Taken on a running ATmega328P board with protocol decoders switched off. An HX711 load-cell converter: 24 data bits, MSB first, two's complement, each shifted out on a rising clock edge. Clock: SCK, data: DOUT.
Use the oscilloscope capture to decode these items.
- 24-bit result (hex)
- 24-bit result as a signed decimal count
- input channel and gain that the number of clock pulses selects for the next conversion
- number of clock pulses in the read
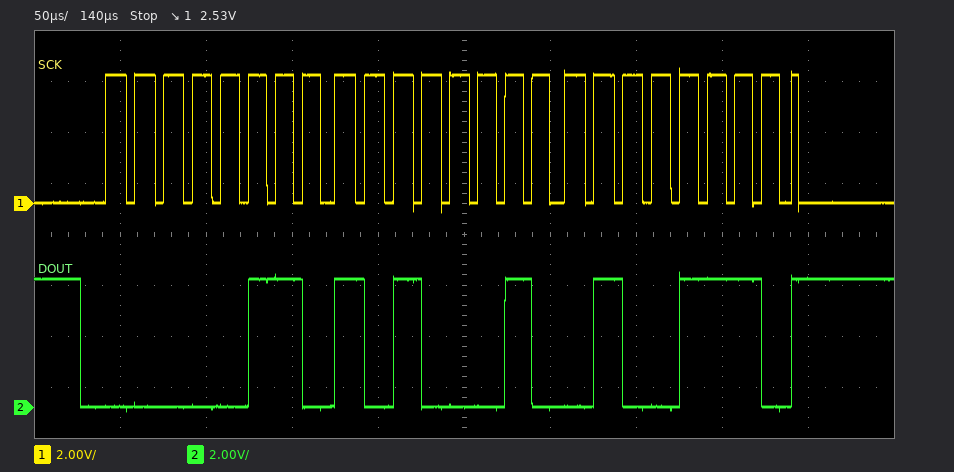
0x06A24E
434766
channel A, gain 128
25
